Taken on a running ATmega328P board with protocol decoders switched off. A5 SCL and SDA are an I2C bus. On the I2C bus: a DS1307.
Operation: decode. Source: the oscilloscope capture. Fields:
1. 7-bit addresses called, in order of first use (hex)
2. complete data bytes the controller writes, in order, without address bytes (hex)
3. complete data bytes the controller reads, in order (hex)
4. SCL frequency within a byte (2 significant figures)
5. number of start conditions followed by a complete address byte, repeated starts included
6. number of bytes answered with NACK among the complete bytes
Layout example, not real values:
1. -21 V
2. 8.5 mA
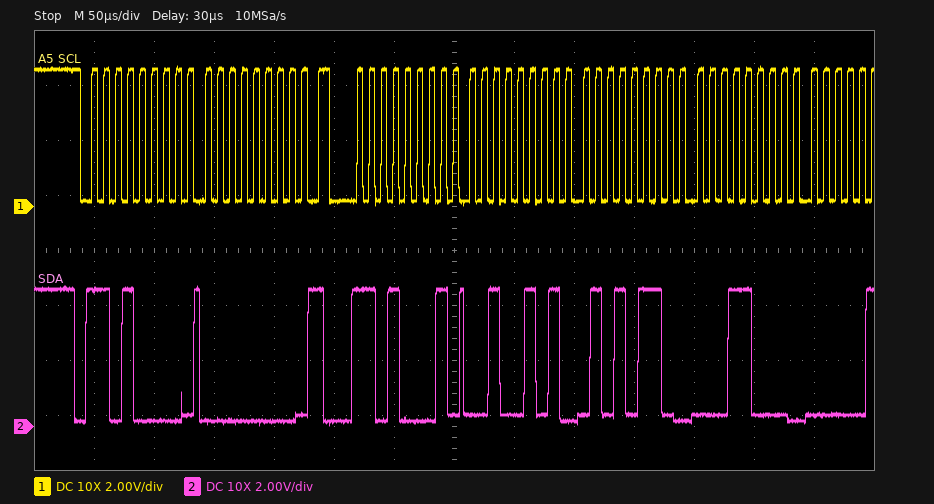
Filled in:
1. 0x68
2. 00
3. 25 56 18
4. 100 kHz
5. 2
6. 0
